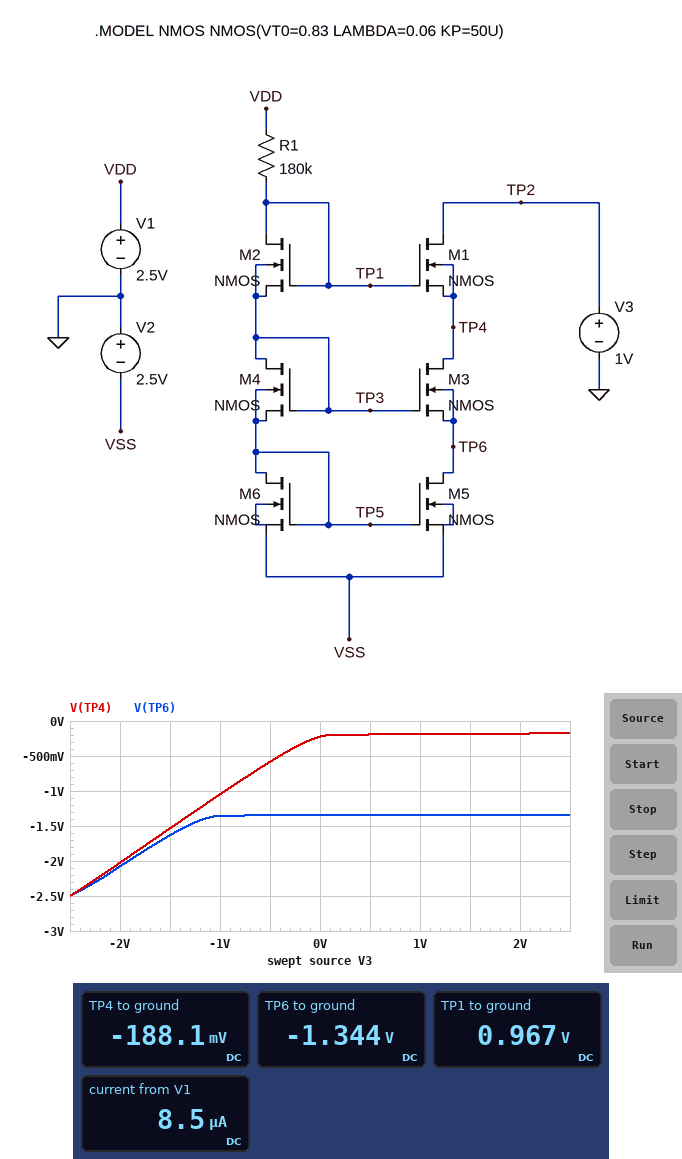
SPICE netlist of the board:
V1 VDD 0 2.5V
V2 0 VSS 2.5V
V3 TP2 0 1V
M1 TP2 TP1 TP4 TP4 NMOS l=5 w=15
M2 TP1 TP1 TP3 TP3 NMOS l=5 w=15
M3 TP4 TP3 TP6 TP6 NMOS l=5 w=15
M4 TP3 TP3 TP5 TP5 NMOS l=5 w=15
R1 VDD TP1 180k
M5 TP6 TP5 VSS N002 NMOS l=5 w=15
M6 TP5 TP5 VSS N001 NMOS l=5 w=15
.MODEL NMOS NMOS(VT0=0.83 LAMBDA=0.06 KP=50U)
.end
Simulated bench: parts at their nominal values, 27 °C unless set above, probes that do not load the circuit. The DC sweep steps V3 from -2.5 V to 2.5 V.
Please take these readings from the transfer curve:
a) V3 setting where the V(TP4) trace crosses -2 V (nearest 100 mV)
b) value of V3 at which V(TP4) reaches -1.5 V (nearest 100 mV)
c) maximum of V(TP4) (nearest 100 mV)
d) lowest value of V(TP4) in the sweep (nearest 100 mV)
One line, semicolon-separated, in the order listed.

-2.0 V; -1.5 V; -200 mV; -2.5 V
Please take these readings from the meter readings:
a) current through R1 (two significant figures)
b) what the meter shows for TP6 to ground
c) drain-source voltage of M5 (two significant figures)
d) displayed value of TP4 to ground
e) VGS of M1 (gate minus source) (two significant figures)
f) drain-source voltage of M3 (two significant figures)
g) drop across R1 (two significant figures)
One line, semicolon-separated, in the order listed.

8.5 µA; -1.344 V; 1.2 V; -188.1 mV; 1.2 V; 1.2 V; 1.5 V
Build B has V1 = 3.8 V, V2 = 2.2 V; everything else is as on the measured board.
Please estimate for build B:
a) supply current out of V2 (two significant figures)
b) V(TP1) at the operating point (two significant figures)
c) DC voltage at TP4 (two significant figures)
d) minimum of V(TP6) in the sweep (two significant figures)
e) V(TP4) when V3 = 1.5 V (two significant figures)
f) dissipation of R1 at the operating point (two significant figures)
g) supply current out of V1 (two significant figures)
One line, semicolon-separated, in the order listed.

26 µA; 1.5 V; 250 mV; -2.4 V; 260 mV; 30 µW; 13 µA
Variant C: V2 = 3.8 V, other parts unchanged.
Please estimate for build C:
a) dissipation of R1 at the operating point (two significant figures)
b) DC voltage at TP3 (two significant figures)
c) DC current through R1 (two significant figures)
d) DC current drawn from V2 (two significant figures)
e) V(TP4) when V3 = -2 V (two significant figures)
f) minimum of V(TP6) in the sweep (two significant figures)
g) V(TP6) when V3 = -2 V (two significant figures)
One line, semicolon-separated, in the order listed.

36 µW; -1.3 V; 14 µA; 28 µA; -2.1 V; -2.7 V; -2.6 V
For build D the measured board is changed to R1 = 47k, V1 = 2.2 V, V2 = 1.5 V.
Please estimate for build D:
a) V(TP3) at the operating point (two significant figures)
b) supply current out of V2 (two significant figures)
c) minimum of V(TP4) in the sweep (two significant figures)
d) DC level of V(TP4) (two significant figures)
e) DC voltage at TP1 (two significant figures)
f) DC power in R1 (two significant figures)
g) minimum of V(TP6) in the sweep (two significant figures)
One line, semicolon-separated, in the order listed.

750 mV; 14 µA; -2.4 V; 740 mV; 1.9 V; 2.3 µW; -2.2 V
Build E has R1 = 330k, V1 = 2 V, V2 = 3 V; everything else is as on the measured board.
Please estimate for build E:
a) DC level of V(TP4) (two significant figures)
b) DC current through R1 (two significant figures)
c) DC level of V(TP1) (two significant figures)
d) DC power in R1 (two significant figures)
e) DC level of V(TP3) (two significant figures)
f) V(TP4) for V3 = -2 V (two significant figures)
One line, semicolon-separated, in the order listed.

-820 mV; 5.3 µA; 260 mV; 9.2 µW; -830 mV; -2.0 V
